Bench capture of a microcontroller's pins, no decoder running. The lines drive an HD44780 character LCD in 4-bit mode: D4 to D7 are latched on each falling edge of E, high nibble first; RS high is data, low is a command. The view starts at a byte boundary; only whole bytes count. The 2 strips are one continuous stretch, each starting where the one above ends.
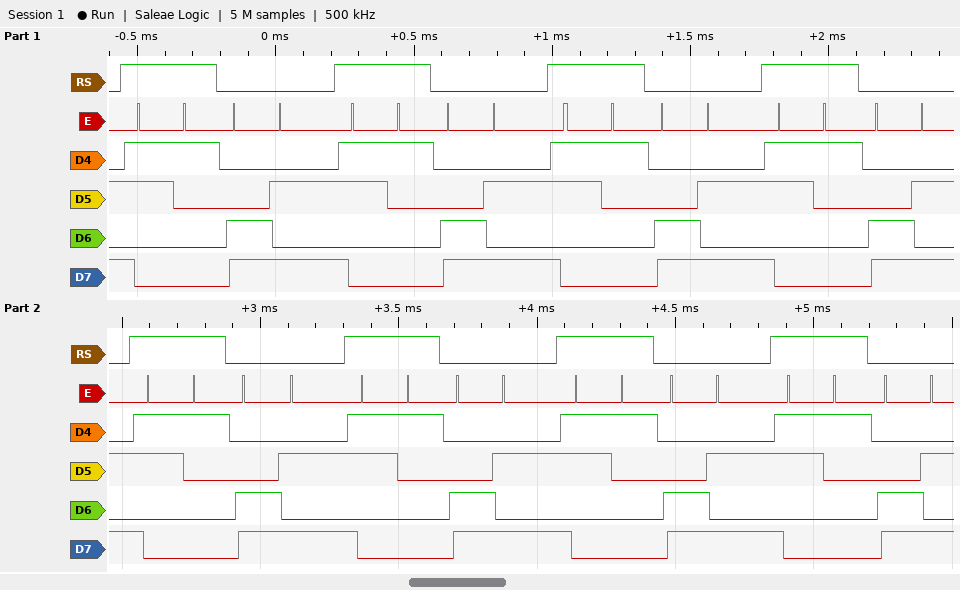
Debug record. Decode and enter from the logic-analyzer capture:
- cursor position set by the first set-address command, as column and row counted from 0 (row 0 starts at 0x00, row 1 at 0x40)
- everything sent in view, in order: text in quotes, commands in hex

column 10, row 1
"1" 0xCA "1" 0xCA "1" 0xCA "1" 0xCA "1" 0xCA "1" 0xCA "1" 0xCA "1" 0xCA
